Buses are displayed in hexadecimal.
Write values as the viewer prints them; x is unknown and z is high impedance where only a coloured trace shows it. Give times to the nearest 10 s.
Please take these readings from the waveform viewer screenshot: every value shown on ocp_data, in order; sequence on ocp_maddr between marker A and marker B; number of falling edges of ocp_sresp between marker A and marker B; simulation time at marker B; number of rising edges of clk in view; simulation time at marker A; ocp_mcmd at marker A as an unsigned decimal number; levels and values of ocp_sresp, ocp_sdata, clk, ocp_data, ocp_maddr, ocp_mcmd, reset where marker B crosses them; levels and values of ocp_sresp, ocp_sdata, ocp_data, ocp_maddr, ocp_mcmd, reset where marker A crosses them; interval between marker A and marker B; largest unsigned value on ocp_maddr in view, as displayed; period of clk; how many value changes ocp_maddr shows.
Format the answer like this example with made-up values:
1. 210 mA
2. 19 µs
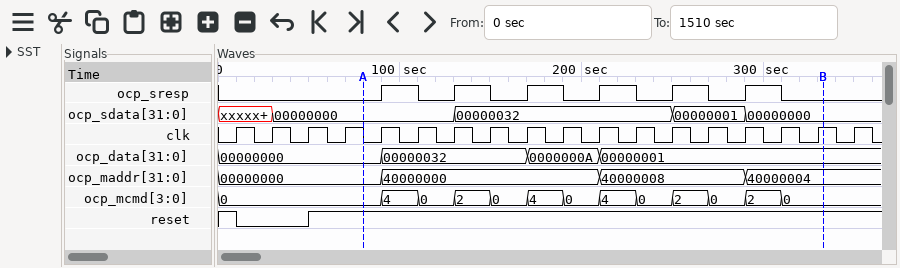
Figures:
1. 00000000, 00000032, 0000000A, 00000001
2. 00000000, 40000000, 40000008, 40000004
3. 6
4. 330 s
5. 18
6. 80 s
7. 0
8. ocp_sresp=0, ocp_sdata=00000000, clk=1, ocp_data=00000001, ocp_maddr=40000004, ocp_mcmd=0, reset=1
9. ocp_sresp=0, ocp_sdata=00000000, ocp_data=00000000, ocp_maddr=00000000, ocp_mcmd=0, reset=1
10. 250 s
11. 40000008
12. 20 s
13. 3
